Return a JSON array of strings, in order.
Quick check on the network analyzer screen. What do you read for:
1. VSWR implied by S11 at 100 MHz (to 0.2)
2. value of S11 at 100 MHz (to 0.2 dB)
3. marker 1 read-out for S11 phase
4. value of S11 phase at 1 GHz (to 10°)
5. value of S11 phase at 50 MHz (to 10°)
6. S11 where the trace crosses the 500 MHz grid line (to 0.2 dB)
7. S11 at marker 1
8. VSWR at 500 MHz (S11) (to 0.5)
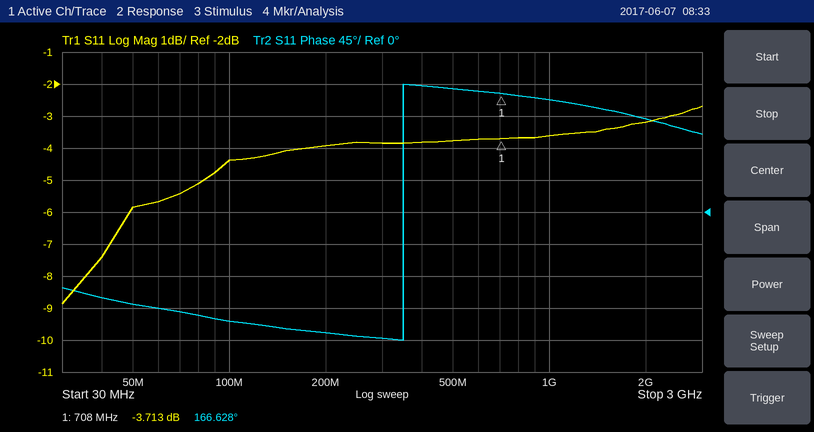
["4.0", "-4.4 dB", "166.628°", "160°", "-130°", "-3.8 dB", "-3.713 dB", "4.5"]
